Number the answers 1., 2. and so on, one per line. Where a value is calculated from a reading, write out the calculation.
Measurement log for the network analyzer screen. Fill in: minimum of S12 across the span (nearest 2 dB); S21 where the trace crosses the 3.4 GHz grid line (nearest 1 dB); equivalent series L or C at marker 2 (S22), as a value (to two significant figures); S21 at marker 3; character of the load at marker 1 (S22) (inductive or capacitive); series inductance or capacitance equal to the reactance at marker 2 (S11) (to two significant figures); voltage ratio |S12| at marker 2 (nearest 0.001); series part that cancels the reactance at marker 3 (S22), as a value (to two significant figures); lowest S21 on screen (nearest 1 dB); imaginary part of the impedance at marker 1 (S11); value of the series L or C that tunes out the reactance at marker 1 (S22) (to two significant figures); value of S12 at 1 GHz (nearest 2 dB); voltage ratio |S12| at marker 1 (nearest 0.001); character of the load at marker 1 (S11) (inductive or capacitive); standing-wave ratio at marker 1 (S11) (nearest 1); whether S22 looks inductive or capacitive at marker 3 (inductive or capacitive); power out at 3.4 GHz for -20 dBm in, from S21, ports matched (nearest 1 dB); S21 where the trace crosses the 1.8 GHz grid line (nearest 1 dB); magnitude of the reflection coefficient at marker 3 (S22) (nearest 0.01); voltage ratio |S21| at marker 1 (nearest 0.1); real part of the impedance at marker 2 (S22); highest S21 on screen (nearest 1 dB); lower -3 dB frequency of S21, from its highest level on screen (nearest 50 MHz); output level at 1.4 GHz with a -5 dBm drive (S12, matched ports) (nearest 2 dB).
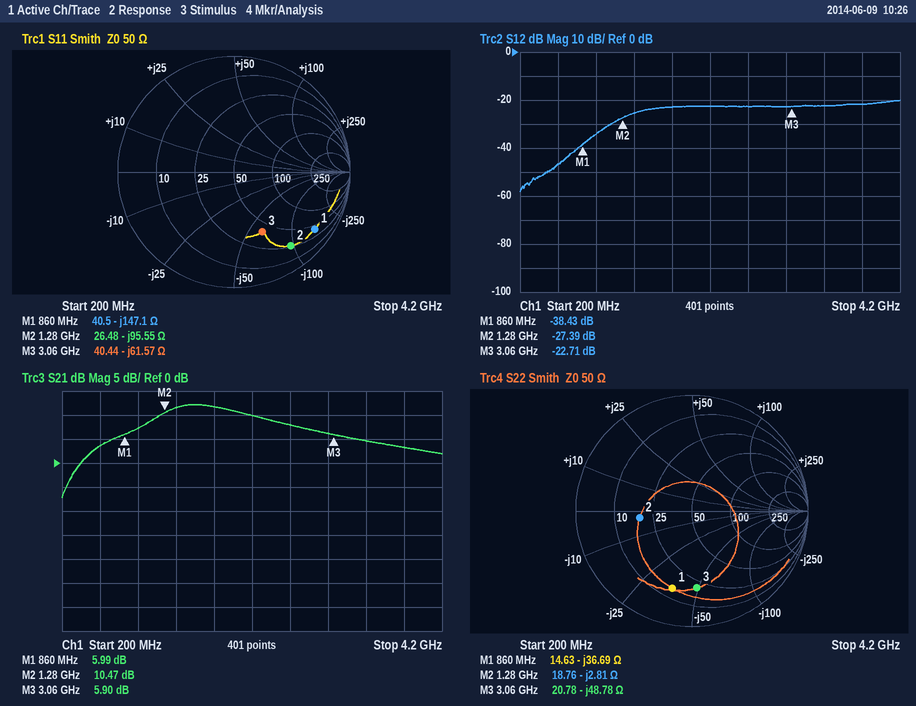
1. -58 dB
2. 5 dB
3. C = 1/(2π × 1.28 GHz × 2.81 Ω) ≈ 44 pF
4. 5.90 dB
5. capacitive
6. C = 1/(2π × 1.28 GHz × 95.55 Ω) ≈ 1.3 pF
7. 10^(-27.39/20) ≈ 0.043
8. L = 48.78 Ω/(2π × 3.06 GHz) ≈ 2.5 nH
9. -7 dB
10. -147.1 Ω
11. L = 36.69 Ω/(2π × 860 MHz) ≈ 6.8 nH
12. -34 dB
13. 10^(-38.43/20) ≈ 0.012
14. capacitive
15. 13
16. capacitive
17. -20 dBm + (5 dB) = -15 dBm
18. 12 dB
19. 0.66
20. 10^(5.99/20) ≈ 2.0
21. 18.76 Ω
22. 12 dB
23. 1.15 GHz
24. -5 dBm + (-26 dB) = -30 dBm
